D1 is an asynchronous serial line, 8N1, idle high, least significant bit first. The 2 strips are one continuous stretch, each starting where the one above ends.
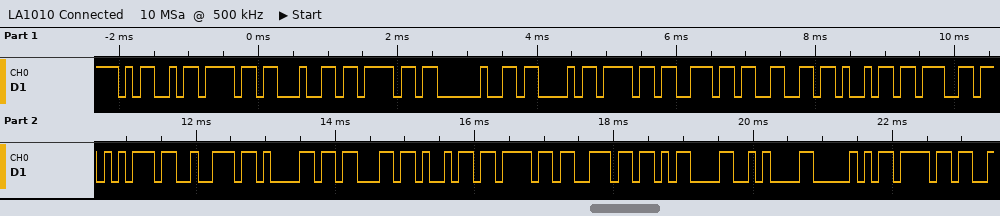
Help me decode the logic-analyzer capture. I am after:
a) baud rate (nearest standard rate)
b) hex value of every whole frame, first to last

9600 baud
0x4D 0x6F 0x64 0x6F 0x20 0x43 0x6F 0x6E 0x66 0x69 0x67 0x75 0x72 0x61 0x63 0x69 0x6F 0x6E 0x0D 0x0A 0x50 0x6F
